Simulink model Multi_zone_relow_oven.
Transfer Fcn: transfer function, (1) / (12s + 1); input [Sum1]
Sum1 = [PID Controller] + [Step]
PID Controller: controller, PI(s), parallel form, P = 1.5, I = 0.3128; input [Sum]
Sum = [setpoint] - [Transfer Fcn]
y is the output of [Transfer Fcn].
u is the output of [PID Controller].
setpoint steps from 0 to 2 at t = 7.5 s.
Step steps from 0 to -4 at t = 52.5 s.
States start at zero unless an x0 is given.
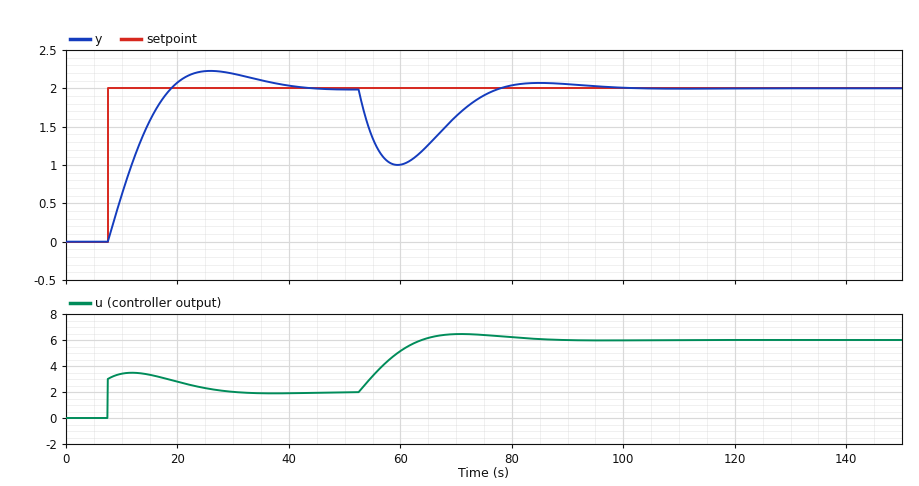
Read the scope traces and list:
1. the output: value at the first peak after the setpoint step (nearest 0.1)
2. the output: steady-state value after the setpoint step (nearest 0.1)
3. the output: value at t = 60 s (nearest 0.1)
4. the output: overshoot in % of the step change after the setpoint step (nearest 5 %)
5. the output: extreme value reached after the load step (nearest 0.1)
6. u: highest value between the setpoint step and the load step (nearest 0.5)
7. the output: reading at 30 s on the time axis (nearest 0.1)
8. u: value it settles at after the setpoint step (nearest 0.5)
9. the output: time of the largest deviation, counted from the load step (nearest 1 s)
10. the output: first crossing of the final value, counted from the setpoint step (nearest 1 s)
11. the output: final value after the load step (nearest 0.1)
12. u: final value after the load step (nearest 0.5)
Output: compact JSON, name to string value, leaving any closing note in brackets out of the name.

{"the output: value at the first peak after the setpoint step": "2.2", "the output: steady-state value after the setpoint step": "2.0", "the output: value at t = 60 s": "1.0", "the output: overshoot in % of the step change after the setpoint step": "10 %", "the output: extreme value reached after the load step": "1.0", "u: highest value between the setpoint step and the load step": "3.5", "the output: reading at 30 s on the time axis": "2.2", "u: value it settles at after the setpoint step": "2.0", "the output: time of the largest deviation, counted from the load step": "7 s", "the output: first crossing of the final value, counted from the setpoint step": "11 s", "the output: final value after the load step": "2.0", "u: final value after the load step": "6.0"}
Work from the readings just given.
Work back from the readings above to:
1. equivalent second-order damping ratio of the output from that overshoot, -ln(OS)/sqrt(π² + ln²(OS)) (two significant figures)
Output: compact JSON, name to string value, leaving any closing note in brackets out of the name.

{"equivalent second-order damping ratio of the output from that overshoot, -ln(OS)/sqrt(π² + ln²(OS))": "0.59"}
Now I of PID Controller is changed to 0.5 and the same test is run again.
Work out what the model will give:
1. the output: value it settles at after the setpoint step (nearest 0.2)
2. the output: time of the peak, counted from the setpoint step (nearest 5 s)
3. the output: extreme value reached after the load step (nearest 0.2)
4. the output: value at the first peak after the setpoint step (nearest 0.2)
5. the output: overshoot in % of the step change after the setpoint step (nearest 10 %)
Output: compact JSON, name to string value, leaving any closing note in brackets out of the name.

{"the output: value it settles at after the setpoint step": "2.0", "the output: time of the peak, counted from the setpoint step": "15 s", "the output: extreme value reached after the load step": "1.2", "the output: value at the first peak after the setpoint step": "2.4", "the output: overshoot in % of the step change after the setpoint step": "20 %"}
